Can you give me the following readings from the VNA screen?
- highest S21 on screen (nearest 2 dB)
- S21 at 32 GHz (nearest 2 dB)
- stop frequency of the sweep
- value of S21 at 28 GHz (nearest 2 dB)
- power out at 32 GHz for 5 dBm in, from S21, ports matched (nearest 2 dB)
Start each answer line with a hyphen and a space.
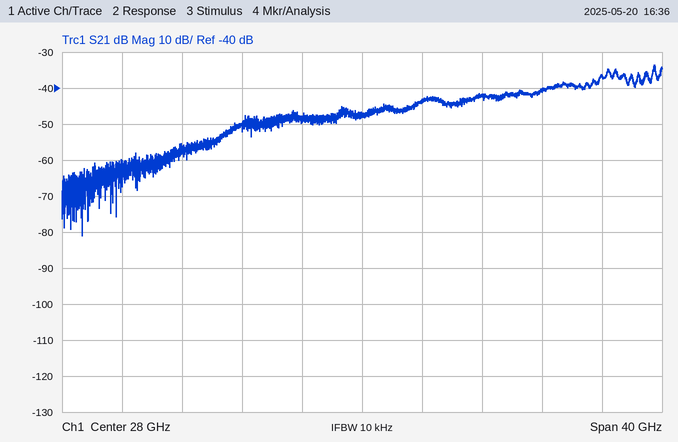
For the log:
- -34 dB
- -44 dB
- 48 GHz
- -48 dB
- -38 dBm
